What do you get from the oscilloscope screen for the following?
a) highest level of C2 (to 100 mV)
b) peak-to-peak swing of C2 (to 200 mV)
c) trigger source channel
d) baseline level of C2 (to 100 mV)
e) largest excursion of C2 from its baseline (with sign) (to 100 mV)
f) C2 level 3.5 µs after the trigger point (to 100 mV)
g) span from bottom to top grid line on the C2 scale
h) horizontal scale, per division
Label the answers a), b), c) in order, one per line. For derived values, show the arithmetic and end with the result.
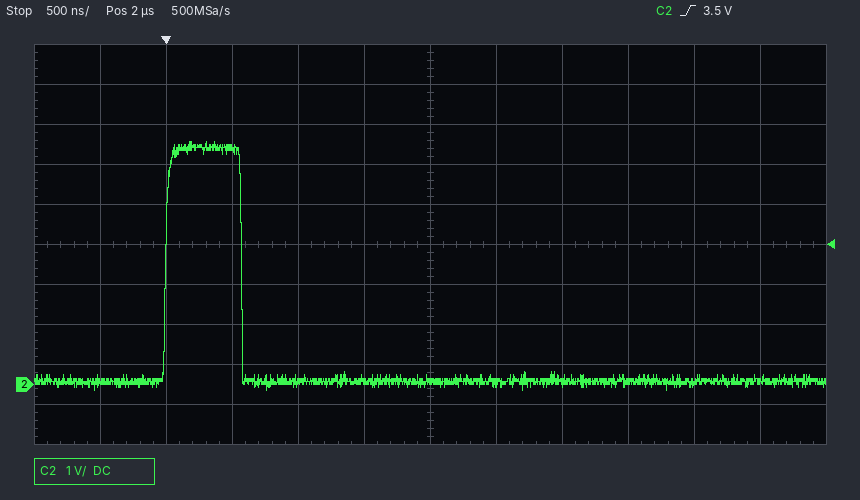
a) 6.1 V
b) 6.2 V
c) C2
d) 100 mV
e) 6.1 V − (100 mV) = +6.0 V
f) 100 mV
g) 10 V
h) 500 ns
